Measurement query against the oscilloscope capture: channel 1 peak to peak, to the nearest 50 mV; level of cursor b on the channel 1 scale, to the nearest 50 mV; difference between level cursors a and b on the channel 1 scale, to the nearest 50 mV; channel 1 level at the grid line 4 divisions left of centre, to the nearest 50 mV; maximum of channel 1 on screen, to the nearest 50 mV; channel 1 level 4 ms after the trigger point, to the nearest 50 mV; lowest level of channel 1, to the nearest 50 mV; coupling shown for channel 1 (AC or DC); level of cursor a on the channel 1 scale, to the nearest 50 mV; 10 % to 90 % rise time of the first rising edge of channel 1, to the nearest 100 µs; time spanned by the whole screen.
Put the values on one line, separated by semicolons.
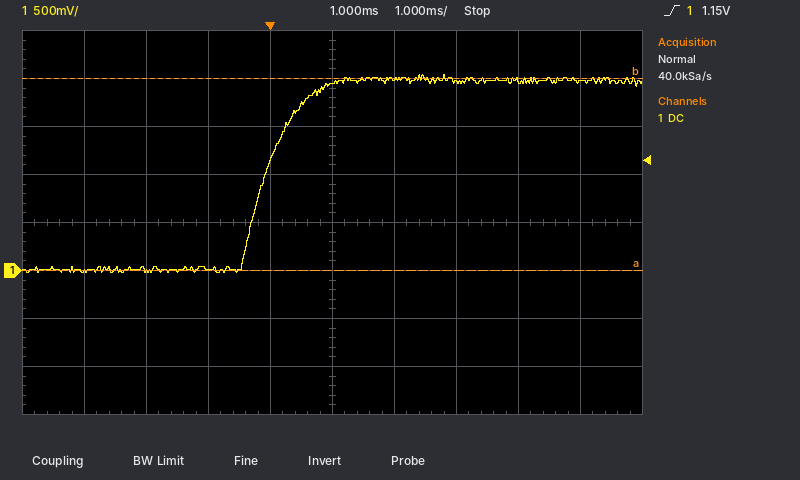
2.05 V; 2.00 V; 2.00 V; 0 mV; 2.05 V; 2.00 V; 0 mV; DC; 0 mV; 1.0 ms; 10 ms
